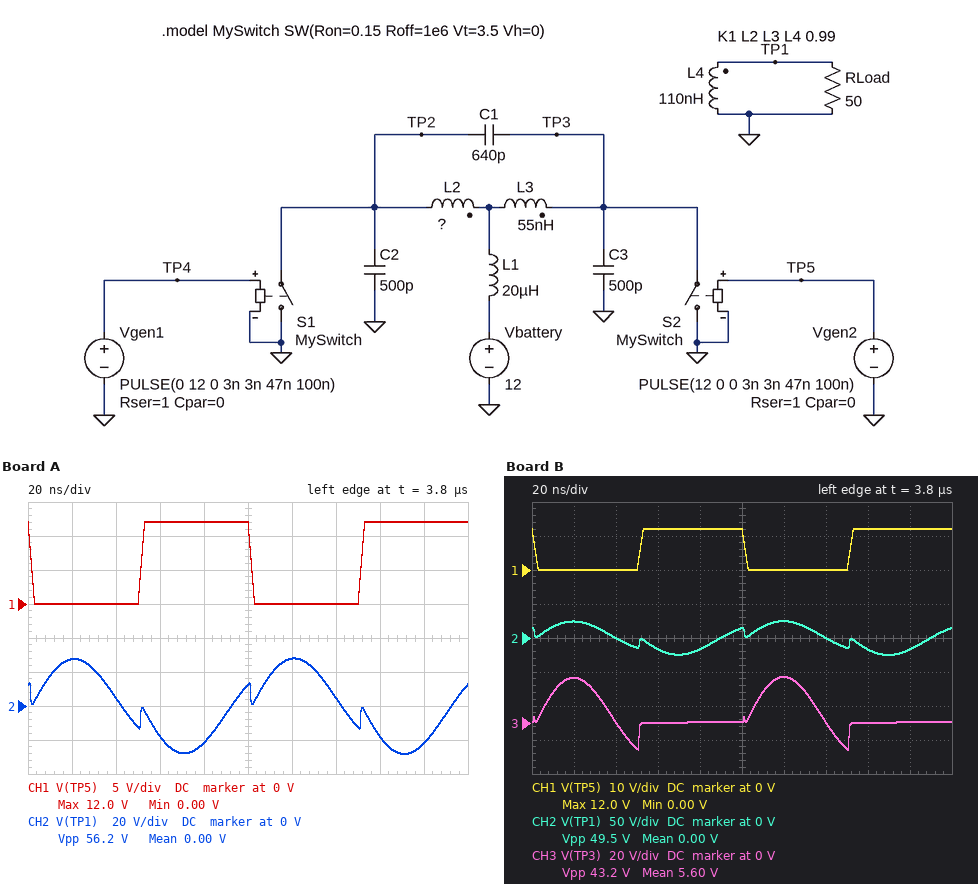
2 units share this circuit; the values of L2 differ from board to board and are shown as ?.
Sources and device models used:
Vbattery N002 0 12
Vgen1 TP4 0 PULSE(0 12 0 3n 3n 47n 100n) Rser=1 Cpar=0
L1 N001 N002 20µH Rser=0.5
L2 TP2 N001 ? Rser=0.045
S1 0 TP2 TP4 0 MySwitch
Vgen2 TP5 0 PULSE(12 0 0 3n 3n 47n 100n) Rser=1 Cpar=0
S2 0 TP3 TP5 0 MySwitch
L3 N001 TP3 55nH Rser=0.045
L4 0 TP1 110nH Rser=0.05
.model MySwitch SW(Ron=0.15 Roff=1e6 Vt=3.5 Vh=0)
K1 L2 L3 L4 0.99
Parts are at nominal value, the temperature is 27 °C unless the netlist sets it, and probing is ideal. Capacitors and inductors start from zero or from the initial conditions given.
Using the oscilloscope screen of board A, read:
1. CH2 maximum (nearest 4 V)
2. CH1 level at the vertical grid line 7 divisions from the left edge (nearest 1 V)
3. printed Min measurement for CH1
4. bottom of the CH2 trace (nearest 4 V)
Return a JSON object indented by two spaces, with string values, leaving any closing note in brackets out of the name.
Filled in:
{
  "CH2 maximum": "28 V",
  "CH1 level at the vertical grid line 7 divisions from the left edge": "0 V",
  "printed Min measurement for CH1": "0.00 V",
  "bottom of the CH2 trace": "-28 V"
}
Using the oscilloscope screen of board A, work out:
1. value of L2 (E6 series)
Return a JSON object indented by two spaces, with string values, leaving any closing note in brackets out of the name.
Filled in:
{
  "value of L2": "22 nH"
}
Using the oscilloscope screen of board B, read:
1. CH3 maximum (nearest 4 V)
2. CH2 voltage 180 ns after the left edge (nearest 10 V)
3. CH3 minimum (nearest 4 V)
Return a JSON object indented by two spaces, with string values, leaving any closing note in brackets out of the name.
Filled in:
{
  "CH3 maximum": "28 V",
  "CH2 voltage 180 ns after the left edge": "-20 V",
  "CH3 minimum": "-16 V"
}
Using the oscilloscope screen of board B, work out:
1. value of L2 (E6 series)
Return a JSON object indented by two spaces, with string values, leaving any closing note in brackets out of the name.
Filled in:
{
  "value of L2": "15 nH"
}
